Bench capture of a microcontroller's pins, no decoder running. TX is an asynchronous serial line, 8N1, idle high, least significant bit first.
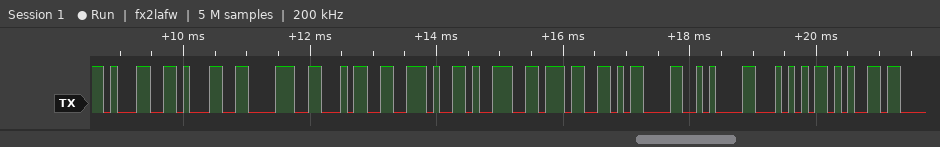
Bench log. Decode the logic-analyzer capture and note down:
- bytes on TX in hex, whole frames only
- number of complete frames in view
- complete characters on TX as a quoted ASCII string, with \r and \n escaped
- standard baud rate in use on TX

31 31 38 34 2E 39 37 0D 0A 54 65
11
"1184.97\r\nTe"
9600 baud
